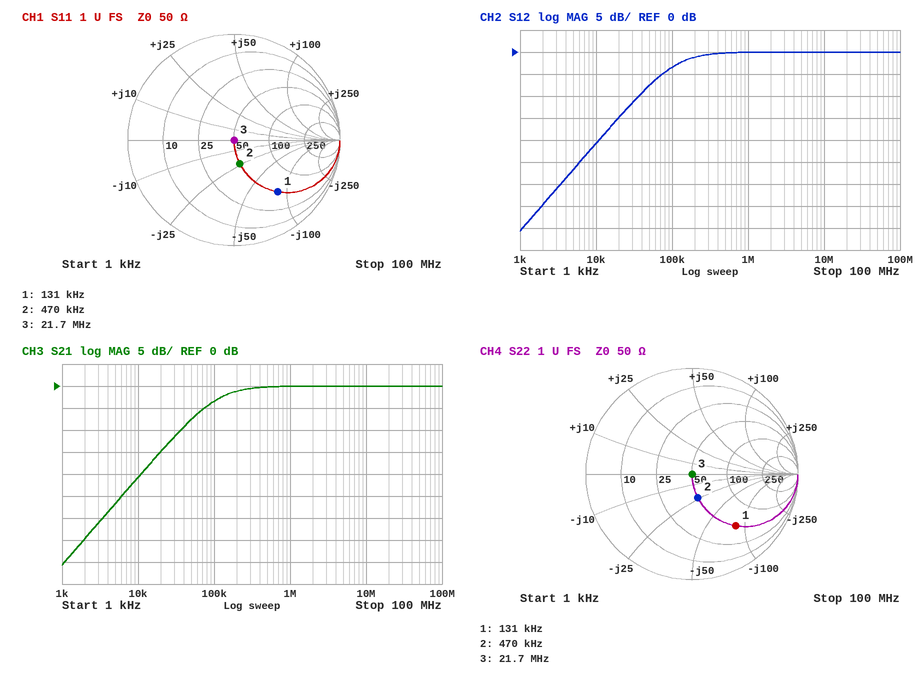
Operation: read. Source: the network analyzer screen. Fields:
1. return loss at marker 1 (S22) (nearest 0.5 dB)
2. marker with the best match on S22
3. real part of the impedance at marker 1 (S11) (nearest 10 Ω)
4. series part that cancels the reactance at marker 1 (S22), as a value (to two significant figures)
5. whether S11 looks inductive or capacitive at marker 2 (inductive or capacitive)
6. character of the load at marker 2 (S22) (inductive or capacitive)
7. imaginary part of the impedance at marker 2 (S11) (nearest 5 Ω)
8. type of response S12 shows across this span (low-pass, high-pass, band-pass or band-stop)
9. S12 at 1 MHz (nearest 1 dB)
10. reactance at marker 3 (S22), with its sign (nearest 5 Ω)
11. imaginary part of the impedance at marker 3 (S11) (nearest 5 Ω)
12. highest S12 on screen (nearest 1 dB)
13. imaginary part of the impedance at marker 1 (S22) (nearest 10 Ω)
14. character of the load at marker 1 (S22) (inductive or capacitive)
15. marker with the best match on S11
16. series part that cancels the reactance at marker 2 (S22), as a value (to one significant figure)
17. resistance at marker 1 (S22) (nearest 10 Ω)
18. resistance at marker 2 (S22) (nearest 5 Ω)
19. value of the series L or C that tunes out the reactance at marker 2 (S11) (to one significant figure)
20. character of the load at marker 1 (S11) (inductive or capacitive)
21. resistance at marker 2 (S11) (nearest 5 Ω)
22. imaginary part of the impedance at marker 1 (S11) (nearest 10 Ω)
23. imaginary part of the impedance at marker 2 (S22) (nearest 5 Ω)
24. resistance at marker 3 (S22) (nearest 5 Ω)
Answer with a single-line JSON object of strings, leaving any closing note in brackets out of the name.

{"return loss at marker 1 (S22)": "4.0 dB", "marker with the best match on S22": "marker 3", "real part of the impedance at marker 1 (S11)": "50 Ω", "series part that cancels the reactance at marker 1 (S22), as a value": "100 µH", "whether S11 looks inductive or capacitive at marker 2": "capacitive", "character of the load at marker 2 (S22)": "capacitive", "imaginary part of the impedance at marker 2 (S11)": "-25 Ω", "type of response S12 shows across this span": "high-pass", "S12 at 1 MHz": "0 dB", "reactance at marker 3 (S22), with its sign": "0 Ω", "imaginary part of the impedance at marker 3 (S11)": "0 Ω", "highest S12 on screen": "0 dB", "imaginary part of the impedance at marker 1 (S22)": "-80 Ω", "character of the load at marker 1 (S22)": "capacitive", "marker with the best match on S11": "marker 3", "series part that cancels the reactance at marker 2 (S22), as a value": "8 µH", "resistance at marker 1 (S22)": "50 Ω", "resistance at marker 2 (S22)": "50 Ω", "value of the series L or C that tunes out the reactance at marker 2 (S11)": "8 µH", "character of the load at marker 1 (S11)": "capacitive", "resistance at marker 2 (S11)": "50 Ω", "imaginary part of the impedance at marker 1 (S11)": "-80 Ω", "imaginary part of the impedance at marker 2 (S22)": "-25 Ω", "resistance at marker 3 (S22)": "50 Ω"}
